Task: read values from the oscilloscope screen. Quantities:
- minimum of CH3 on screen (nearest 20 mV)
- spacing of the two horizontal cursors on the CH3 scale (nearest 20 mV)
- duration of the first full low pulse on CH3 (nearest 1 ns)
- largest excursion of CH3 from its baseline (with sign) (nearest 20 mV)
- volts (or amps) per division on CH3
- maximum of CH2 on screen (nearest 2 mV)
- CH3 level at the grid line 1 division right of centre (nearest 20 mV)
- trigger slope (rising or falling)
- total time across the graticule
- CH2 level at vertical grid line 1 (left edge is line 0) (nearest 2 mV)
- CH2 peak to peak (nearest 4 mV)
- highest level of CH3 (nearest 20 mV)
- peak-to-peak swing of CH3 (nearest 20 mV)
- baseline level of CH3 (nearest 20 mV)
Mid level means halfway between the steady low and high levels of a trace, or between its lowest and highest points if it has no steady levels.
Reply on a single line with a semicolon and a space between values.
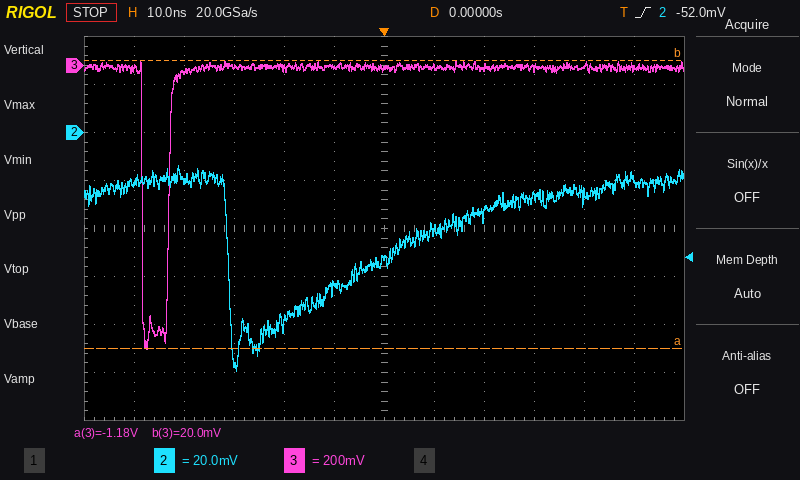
-1.18 V; 1.20 V; 5 ns; -1.18 V; 200 mV; -14 mV; 0 mV; rising; 120 ns; -20 mV; 84 mV; 20 mV; 1.20 V; 0 mV
